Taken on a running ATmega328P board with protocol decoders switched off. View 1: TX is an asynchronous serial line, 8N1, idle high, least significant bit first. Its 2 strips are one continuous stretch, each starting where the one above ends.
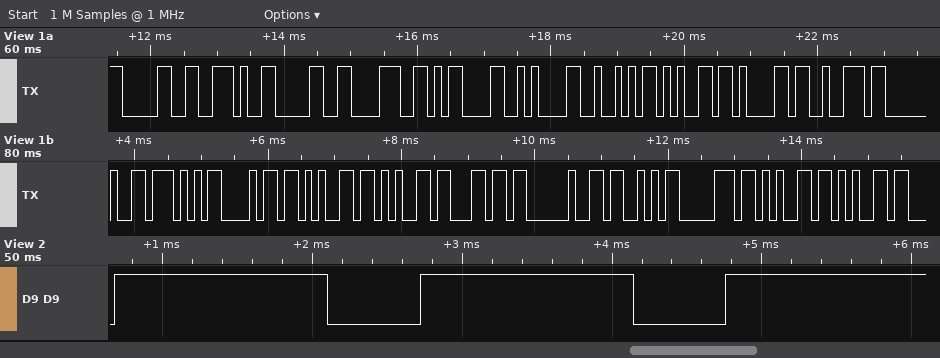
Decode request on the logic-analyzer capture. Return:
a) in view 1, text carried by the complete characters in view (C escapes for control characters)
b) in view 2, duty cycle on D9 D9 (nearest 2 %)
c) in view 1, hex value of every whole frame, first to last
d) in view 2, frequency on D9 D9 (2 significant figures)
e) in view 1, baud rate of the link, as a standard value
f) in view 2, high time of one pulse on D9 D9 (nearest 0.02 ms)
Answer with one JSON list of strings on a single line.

["\"0.08\\r\\nRear Wheel Spee\"", "70 %", "0x30 0x2E 0x30 0x38 0x0D 0x0A 0x52 0x65 0x61 0x72 0x20 0x57 0x68 0x65 0x65 0x6C 0x20 0x53 0x70 0x65 0x65", "490 Hz", "9600 baud", "1.42 ms"]
